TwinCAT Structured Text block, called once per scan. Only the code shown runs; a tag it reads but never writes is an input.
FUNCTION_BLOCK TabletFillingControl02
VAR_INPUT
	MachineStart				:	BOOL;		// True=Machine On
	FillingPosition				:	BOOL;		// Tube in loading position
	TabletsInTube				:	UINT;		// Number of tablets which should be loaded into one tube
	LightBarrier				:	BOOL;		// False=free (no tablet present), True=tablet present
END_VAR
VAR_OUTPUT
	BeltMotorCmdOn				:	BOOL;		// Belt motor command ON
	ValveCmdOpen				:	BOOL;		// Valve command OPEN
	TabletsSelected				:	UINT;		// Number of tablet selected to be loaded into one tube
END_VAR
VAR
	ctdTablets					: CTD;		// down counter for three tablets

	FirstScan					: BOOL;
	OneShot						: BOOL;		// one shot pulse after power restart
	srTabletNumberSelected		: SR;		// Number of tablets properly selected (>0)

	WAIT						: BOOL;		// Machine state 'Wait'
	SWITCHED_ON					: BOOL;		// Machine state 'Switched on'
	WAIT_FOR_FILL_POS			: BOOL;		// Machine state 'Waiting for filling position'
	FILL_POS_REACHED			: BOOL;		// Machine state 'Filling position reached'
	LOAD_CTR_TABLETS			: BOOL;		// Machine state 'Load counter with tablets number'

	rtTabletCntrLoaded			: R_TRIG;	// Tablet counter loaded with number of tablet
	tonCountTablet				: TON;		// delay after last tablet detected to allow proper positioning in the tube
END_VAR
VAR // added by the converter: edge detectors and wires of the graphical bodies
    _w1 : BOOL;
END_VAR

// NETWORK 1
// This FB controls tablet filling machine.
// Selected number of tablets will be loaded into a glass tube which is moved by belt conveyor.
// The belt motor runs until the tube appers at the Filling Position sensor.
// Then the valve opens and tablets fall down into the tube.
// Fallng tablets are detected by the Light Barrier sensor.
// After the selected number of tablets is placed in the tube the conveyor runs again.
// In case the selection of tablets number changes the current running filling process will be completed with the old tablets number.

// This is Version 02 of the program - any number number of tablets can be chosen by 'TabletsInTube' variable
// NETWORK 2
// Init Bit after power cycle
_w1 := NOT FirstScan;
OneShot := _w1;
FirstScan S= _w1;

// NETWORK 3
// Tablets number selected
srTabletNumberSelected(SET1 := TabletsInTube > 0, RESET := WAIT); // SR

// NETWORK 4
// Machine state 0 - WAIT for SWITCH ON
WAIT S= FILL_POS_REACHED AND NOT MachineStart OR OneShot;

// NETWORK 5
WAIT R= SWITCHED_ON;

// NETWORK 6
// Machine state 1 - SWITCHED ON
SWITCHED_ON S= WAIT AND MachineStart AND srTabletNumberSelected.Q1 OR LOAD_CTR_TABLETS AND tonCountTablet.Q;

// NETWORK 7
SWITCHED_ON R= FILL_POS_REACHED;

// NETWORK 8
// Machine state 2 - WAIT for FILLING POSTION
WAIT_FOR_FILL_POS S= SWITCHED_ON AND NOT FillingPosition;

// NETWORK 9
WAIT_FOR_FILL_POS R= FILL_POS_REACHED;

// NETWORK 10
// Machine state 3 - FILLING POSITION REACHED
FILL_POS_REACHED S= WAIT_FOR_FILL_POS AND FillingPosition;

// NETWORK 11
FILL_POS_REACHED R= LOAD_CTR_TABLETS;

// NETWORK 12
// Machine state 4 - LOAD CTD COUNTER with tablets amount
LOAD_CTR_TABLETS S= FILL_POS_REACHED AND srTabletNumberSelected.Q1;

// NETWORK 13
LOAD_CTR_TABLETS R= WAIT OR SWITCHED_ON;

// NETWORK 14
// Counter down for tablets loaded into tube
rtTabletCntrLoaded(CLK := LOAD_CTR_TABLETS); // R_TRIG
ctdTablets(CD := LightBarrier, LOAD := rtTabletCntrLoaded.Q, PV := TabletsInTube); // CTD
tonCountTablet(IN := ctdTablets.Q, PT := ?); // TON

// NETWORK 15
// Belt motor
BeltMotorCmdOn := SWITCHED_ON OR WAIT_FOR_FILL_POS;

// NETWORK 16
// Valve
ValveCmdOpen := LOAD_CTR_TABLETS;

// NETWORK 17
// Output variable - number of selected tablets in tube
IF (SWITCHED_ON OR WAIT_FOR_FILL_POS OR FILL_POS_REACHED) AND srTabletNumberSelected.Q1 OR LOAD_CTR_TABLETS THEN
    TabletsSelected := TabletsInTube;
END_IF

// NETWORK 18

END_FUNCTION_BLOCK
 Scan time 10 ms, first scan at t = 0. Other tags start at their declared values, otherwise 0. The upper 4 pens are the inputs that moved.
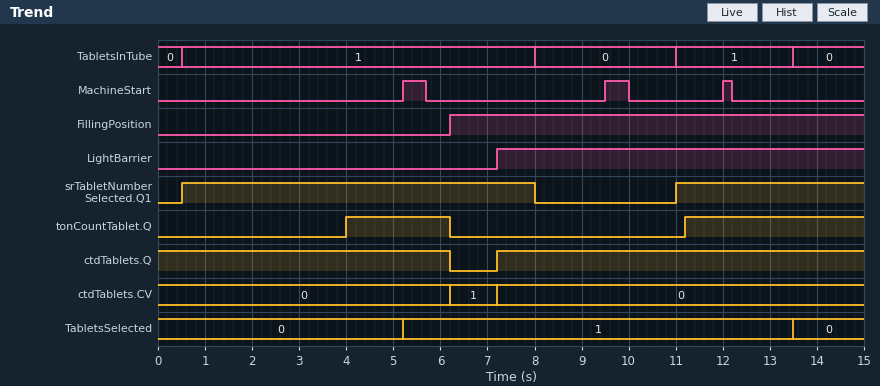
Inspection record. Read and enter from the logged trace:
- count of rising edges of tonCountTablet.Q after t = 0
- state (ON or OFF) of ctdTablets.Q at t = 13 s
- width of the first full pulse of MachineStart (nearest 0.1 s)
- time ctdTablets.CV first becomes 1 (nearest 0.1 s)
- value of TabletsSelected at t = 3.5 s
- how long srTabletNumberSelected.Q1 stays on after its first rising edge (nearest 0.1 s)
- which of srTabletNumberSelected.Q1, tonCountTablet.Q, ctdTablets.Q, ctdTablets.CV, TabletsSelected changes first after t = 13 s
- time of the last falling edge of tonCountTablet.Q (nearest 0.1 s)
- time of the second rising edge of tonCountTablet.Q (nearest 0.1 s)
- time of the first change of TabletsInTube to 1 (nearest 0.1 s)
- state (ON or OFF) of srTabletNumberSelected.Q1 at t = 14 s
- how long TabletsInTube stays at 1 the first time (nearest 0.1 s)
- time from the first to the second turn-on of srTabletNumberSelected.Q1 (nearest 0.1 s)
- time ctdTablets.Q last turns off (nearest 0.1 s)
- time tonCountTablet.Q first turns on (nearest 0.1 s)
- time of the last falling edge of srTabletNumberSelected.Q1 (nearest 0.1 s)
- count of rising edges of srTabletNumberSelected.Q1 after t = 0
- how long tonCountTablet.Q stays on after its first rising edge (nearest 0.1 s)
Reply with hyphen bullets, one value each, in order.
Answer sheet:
- 2
- ON
- 0.5 s
- 6.2 s
- 0
- 7.5 s
- TabletsSelected
- 6.2 s
- 11.2 s
- 0.5 s
- ON
- 7.5 s
- 10.5 s
- 6.2 s
- 4.0 s
- 8.0 s
- 2
- 2.2 s
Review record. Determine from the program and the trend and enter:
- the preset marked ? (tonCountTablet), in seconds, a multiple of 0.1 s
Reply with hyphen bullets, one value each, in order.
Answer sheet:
- 4.0 s
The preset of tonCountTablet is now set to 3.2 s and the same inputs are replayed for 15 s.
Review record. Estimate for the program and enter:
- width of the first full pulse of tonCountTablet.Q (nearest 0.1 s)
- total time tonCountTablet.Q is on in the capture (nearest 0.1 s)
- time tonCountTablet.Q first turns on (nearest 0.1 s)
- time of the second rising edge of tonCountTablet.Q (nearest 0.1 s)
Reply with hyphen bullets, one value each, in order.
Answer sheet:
- 3.0 s
- 7.6 s
- 3.2 s
- 10.4 s
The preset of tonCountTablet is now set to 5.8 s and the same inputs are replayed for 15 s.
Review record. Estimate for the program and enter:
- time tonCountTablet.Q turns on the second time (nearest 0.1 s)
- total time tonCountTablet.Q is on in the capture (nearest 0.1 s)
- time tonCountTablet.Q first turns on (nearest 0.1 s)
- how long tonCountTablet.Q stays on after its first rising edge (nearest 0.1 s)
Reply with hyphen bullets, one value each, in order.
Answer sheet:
- 13.0 s
- 2.4 s
- 5.8 s
- 0.4 s
